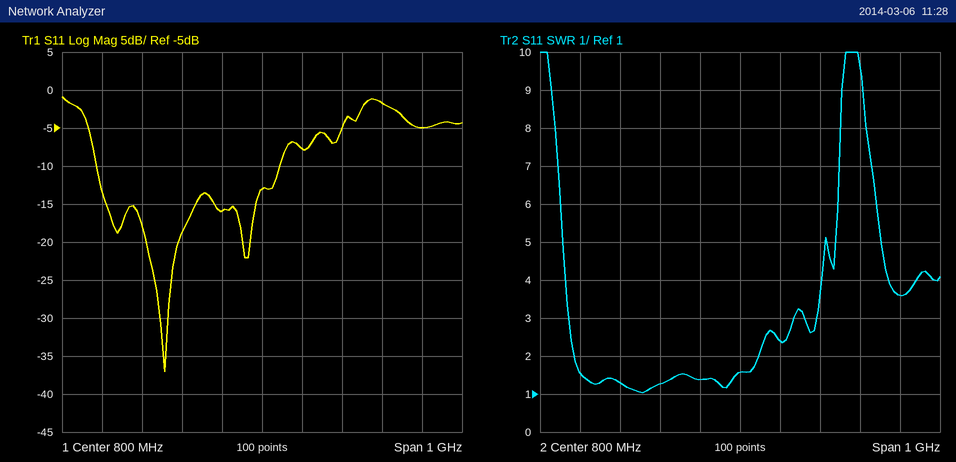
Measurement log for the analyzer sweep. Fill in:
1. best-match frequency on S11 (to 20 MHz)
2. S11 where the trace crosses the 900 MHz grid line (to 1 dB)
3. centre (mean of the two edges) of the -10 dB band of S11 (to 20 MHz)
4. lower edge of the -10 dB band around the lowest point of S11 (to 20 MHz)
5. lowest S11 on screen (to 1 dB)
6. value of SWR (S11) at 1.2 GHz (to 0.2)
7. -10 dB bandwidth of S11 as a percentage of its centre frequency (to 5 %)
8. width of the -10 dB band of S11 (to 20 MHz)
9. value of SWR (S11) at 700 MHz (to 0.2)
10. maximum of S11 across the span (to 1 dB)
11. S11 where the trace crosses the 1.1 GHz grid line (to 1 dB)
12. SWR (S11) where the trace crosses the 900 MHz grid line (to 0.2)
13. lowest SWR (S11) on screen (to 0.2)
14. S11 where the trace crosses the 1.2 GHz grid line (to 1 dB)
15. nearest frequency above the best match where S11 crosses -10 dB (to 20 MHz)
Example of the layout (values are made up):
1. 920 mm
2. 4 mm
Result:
1. 560 MHz
2. -8 dB
3. 620 MHz
4. 380 MHz
5. -37 dB
6. 3.6
7. 75 %
8. 460 MHz
9. 1.4
10. -1 dB
11. -2 dB
12. 2.4
13. 1.0
14. -5 dB
15. 840 MHz
